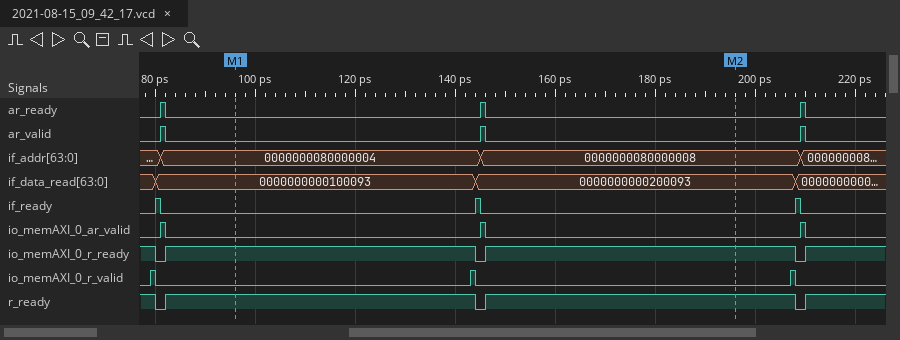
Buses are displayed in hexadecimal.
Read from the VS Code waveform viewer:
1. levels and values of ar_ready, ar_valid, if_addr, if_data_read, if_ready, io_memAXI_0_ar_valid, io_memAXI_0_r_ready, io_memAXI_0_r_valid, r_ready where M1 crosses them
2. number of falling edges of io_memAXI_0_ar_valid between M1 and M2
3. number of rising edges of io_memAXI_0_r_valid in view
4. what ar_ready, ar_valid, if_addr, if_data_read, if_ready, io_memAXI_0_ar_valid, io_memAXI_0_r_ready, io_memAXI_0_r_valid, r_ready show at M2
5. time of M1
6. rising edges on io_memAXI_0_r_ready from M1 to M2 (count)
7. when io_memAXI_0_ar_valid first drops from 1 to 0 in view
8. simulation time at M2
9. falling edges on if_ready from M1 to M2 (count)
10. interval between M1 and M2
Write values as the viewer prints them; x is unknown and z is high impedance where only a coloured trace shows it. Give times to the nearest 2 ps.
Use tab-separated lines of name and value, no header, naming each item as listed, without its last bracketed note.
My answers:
levels and values of ar_ready, ar_valid, if_addr, if_data_read, if_ready, io_memAXI_0_ar_valid, io_memAXI_0_r_ready, io_memAXI_0_r_valid, r_ready where M1 crosses them	ar_ready=0, ar_valid=0, if_addr=0000000080000004, if_data_read=0000000000100093, if_ready=0, io_memAXI_0_ar_valid=0, io_memAXI_0_r_ready=1, io_memAXI_0_r_valid=0, r_ready=1
number of falling edges of io_memAXI_0_ar_valid between M1 and M2	1
number of rising edges of io_memAXI_0_r_valid in view	3
what ar_ready, ar_valid, if_addr, if_data_read, if_ready, io_memAXI_0_ar_valid, io_memAXI_0_r_ready, io_memAXI_0_r_valid, r_ready show at M2	ar_ready=0, ar_valid=0, if_addr=0000000080000008, if_data_read=0000000000200093, if_ready=0, io_memAXI_0_ar_valid=0, io_memAXI_0_r_ready=1, io_memAXI_0_r_valid=0, r_ready=1
time of M1	96 ps
rising edges on io_memAXI_0_r_ready from M1 to M2	1
when io_memAXI_0_ar_valid first drops from 1 to 0 in view	82 ps
simulation time at M2	196 ps
falling edges on if_ready from M1 to M2	1
interval between M1 and M2	100 ps
